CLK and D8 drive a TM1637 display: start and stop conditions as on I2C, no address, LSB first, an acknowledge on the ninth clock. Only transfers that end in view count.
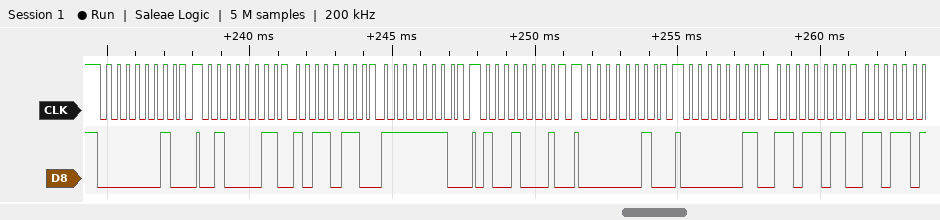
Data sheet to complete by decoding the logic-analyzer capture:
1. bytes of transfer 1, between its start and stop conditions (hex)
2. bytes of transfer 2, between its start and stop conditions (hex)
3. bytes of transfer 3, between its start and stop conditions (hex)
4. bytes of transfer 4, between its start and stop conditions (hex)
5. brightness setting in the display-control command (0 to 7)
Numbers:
40
C2 6D 7F
89
40
1
